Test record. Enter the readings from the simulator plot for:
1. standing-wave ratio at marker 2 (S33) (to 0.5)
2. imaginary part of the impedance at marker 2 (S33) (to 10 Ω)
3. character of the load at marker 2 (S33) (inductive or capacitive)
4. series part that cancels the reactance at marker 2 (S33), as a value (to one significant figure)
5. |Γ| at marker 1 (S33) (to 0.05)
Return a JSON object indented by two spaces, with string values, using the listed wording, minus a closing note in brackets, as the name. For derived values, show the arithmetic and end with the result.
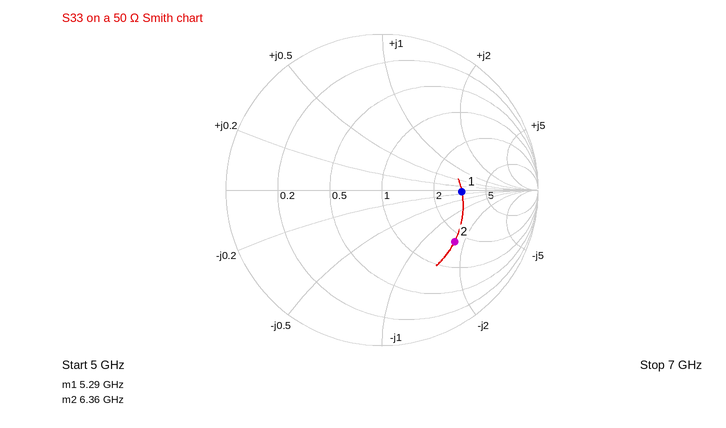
{
  "standing-wave ratio at marker 2 (S33)": "3.5",
  "imaginary part of the impedance at marker 2 (S33)": "-80 Ω",
  "character of the load at marker 2 (S33)": "capacitive",
  "series part that cancels the reactance at marker 2 (S33), as a value": "L = 80 Ω/(2π × 6.36 GHz) ≈ 2 nH",
  "|Γ| at marker 1 (S33)": "0.50"
}
